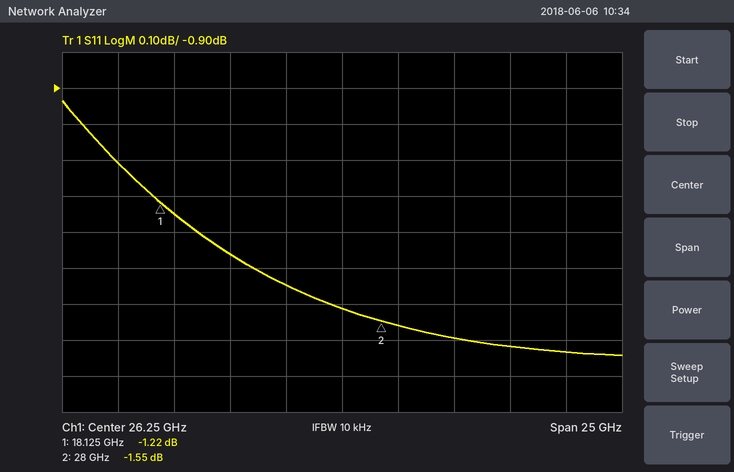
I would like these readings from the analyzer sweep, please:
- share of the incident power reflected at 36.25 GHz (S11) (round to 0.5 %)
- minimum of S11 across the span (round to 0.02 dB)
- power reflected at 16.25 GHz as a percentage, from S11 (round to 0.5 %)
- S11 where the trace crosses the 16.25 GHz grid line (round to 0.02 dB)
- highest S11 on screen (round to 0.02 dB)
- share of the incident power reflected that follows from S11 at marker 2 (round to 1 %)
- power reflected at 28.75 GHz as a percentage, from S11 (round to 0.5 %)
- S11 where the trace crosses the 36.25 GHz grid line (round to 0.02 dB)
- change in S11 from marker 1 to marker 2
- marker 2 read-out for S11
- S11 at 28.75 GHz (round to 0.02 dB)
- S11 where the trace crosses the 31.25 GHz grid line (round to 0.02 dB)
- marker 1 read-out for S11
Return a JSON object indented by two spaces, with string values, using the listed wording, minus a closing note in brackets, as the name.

{
  "share of the incident power reflected at 36.25 GHz (S11)": "68.5 %",
  "minimum of S11 across the span": "-1.64 dB",
  "power reflected at 16.25 GHz as a percentage, from S11": "77.5 %",
  "S11 where the trace crosses the 16.25 GHz grid line": "-1.10 dB",
  "highest S11 on screen": "-0.94 dB",
  "share of the incident power reflected that follows from S11 at marker 2": "70 %",
  "power reflected at 28.75 GHz as a percentage, from S11": "70.0 %",
  "S11 where the trace crosses the 36.25 GHz grid line": "-1.64 dB",
  "change in S11 from marker 1 to marker 2": "-0.33 dB",
  "marker 2 read-out for S11": "-1.55 dB",
  "S11 at 28.75 GHz": "-1.56 dB",
  "S11 where the trace crosses the 31.25 GHz grid line": "-1.60 dB",
  "marker 1 read-out for S11": "-1.22 dB"
}
